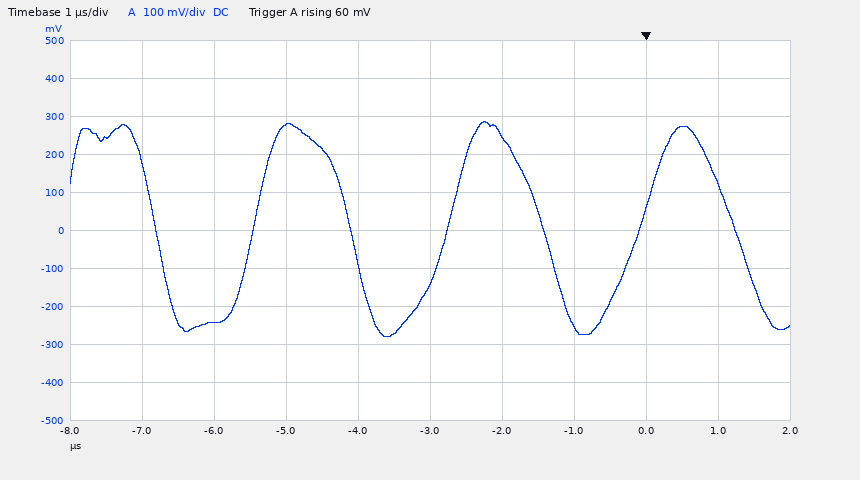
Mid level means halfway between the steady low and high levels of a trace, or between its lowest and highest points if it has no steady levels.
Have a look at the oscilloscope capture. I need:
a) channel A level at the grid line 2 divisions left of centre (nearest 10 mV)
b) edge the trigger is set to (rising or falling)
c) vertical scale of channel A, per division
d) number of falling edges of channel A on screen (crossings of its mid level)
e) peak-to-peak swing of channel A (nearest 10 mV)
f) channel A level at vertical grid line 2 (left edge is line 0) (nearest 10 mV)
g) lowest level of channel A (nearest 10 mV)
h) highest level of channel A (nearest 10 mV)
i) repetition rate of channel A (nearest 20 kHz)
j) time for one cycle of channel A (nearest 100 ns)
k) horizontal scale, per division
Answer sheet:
280 mV
rising
100 mV
4
570 mV
-240 mV
-280 mV
290 mV
380 kHz
2.7 µs
1 µs
